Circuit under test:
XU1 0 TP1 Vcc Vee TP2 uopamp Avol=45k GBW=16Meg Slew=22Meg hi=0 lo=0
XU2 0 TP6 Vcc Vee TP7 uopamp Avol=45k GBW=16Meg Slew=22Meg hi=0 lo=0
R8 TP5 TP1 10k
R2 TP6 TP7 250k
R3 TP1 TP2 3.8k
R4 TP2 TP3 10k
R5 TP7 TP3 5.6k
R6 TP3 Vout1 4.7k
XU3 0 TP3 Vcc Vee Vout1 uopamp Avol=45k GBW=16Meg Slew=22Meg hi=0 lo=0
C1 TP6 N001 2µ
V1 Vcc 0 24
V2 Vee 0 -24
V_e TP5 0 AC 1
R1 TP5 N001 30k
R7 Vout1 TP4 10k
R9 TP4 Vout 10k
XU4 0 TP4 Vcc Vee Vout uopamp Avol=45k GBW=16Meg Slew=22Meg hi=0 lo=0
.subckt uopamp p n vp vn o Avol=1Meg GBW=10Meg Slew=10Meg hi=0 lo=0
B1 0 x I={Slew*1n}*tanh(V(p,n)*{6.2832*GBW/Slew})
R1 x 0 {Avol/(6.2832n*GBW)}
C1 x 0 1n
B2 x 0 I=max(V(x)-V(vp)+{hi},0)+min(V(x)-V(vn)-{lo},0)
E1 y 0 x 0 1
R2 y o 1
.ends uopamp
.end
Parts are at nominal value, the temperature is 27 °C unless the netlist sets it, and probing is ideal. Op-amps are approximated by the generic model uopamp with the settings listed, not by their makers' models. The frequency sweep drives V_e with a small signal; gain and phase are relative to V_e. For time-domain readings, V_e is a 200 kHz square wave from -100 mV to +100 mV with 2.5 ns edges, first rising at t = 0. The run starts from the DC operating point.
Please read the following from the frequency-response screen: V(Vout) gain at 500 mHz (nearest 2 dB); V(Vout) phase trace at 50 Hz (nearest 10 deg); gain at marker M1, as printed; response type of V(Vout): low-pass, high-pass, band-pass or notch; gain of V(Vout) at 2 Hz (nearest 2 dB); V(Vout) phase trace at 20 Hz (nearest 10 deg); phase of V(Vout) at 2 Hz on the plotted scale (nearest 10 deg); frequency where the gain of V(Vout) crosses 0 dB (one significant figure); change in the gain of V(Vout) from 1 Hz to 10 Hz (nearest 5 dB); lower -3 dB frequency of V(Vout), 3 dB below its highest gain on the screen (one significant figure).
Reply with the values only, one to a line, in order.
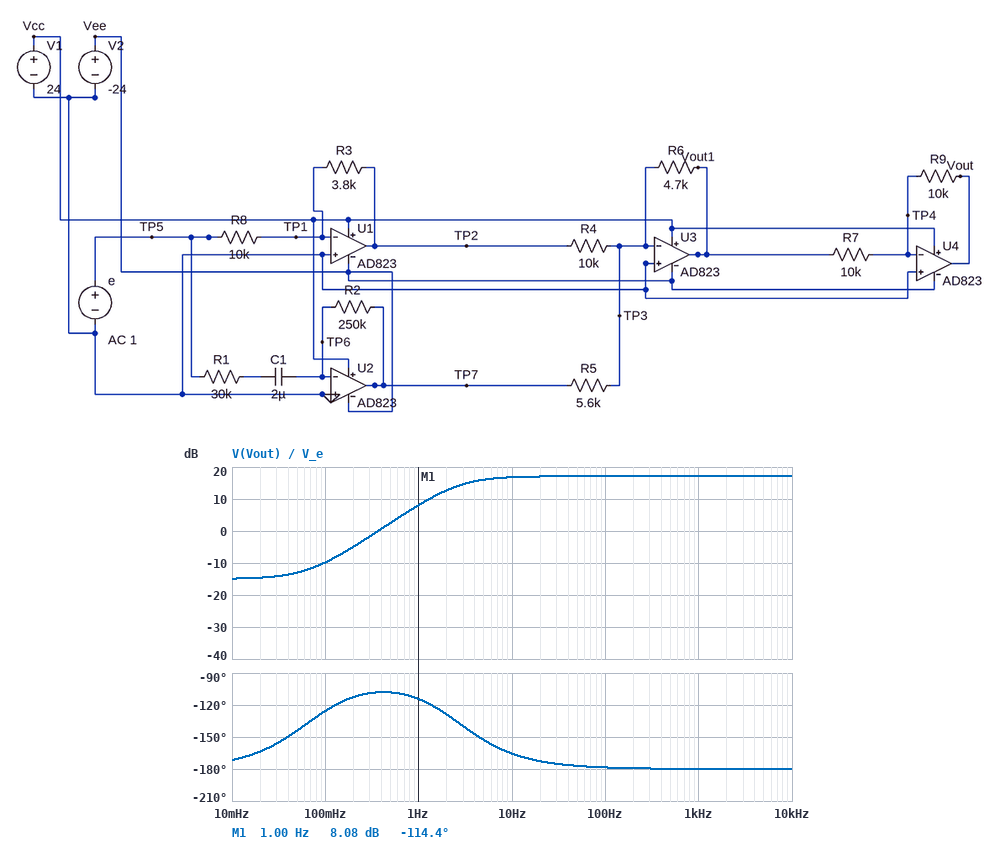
2 dB
-180 deg
8.08 dB
high-pass
12 dB
-170 deg
-130 deg
400 mHz
10 dB
3 Hz
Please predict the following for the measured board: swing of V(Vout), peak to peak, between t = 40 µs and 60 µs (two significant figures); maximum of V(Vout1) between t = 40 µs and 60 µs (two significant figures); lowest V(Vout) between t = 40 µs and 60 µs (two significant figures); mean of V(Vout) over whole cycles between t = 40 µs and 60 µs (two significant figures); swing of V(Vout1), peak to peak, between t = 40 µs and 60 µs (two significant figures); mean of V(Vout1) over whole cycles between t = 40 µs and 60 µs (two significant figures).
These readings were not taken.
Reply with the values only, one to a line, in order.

1.4 V
1.4 V
-1.4 V
-700 mV
1.4 V
700 mV
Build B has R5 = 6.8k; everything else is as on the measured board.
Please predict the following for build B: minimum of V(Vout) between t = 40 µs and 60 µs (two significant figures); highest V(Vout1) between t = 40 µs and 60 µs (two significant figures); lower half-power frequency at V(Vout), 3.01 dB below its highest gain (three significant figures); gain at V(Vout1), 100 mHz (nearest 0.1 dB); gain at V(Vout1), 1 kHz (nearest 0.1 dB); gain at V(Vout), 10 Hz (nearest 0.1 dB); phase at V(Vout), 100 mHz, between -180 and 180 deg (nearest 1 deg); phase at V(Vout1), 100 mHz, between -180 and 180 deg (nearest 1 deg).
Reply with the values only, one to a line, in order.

-1.2 V
1.2 V
2.65 Hz
-10.9 dB
15.5 dB
15.2 dB
-131 deg
49 deg
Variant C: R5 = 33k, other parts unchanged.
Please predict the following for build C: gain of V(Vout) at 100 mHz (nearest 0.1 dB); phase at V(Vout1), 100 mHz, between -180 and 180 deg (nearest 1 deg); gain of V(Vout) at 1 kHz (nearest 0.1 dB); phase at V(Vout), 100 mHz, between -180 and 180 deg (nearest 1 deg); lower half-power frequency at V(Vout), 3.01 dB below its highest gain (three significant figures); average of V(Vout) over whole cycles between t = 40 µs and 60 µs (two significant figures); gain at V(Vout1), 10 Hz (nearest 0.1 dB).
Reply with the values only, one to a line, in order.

-14.6 dB
14 deg
2.7 dB
-166 deg
2.61 Hz
-120 mV
2.4 dB
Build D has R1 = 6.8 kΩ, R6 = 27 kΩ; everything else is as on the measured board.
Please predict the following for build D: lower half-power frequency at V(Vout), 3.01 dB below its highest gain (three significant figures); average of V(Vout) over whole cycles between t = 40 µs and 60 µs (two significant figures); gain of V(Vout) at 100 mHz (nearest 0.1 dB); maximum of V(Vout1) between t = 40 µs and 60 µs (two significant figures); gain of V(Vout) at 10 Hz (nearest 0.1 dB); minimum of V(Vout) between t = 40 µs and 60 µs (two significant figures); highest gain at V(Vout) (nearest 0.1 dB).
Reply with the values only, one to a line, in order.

11.7 Hz
-13 V
5.3 dB
24 V
41.3 dB
-24 V
45.0 dB
